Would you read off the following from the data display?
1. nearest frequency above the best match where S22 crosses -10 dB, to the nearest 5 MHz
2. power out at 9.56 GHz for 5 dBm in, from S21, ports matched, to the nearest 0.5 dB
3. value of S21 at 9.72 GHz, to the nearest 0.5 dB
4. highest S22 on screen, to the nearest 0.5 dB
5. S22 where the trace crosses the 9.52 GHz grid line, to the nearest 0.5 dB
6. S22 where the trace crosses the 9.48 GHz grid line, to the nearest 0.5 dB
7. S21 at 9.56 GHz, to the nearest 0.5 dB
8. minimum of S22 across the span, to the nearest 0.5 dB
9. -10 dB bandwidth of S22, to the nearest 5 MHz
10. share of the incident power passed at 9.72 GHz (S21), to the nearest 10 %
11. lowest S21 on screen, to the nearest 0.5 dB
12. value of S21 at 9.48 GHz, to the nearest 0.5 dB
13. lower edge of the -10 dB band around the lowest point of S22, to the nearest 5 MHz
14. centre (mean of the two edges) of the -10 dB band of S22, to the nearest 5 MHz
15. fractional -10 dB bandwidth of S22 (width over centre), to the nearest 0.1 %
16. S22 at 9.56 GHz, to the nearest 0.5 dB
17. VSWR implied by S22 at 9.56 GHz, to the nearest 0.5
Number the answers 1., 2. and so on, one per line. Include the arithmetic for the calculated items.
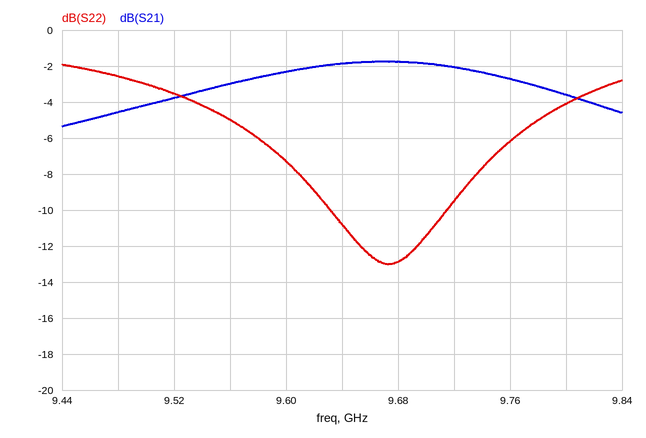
1. 9.715 GHz
2. 5 dBm + (-3.0 dB) = 2.0 dBm
3. -2.0 dB
4. -2.0 dB
5. -3.5 dB
6. -2.5 dB
7. -3.0 dB
8. -13.0 dB
9. 9.715 GHz − 9.630 GHz = 85 MHz
10. 10^(-2/10) ≈ 63.1 %, so 60 % to the nearest 10 %
11. -5.5 dB
12. -4.5 dB
13. 9.630 GHz
14. 9.675 GHz
15. 85 MHz / 9.6725 GHz ≈ 0.9 %
16. -5.0 dB
17. |Γ| = 10^(-5/20) = 0.5623; VSWR = (1 + 0.5623)/(1 − 0.5623) ≈ 3.57, so 3.5 to the nearest 0.5
